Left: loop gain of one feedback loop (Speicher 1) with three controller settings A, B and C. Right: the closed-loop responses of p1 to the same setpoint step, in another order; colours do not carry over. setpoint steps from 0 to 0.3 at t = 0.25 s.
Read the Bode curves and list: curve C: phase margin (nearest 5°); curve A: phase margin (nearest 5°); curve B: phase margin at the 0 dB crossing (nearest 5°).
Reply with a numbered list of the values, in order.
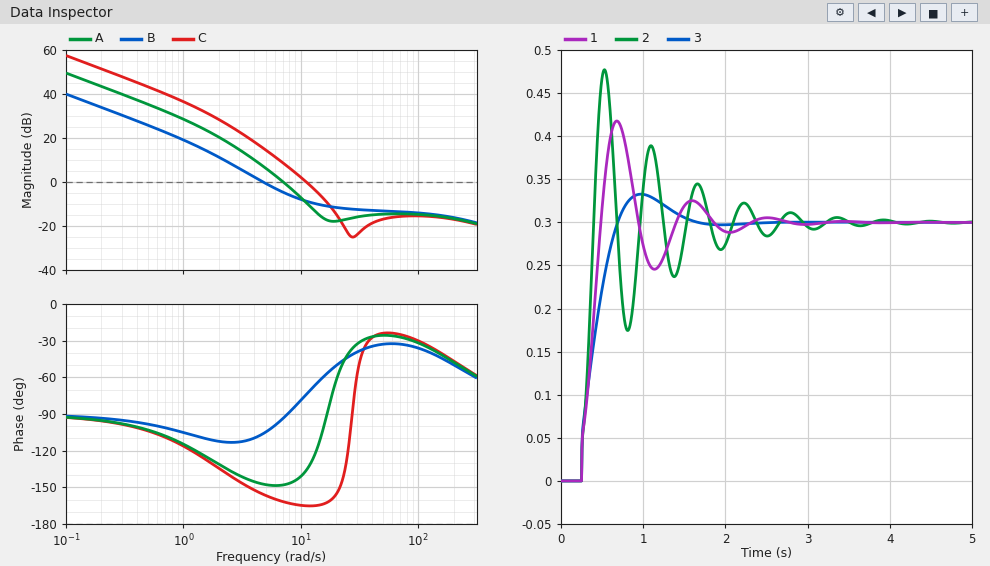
1. 15°
2. 30°
3. 75°
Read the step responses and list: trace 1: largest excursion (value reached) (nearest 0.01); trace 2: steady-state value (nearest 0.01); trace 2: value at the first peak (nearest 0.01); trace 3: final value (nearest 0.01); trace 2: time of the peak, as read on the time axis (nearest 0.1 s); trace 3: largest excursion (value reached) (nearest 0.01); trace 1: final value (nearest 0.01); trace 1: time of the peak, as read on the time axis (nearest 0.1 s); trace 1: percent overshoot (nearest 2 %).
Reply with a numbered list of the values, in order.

1. 0.42
2. 0.30
3. 0.48
4. 0.30
5. 0.5 s
6. 0.33
7. 0.30
8. 0.7 s
9. 40 %
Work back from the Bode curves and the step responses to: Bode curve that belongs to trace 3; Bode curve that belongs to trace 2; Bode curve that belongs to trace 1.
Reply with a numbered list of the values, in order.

1. B
2. C
3. A
